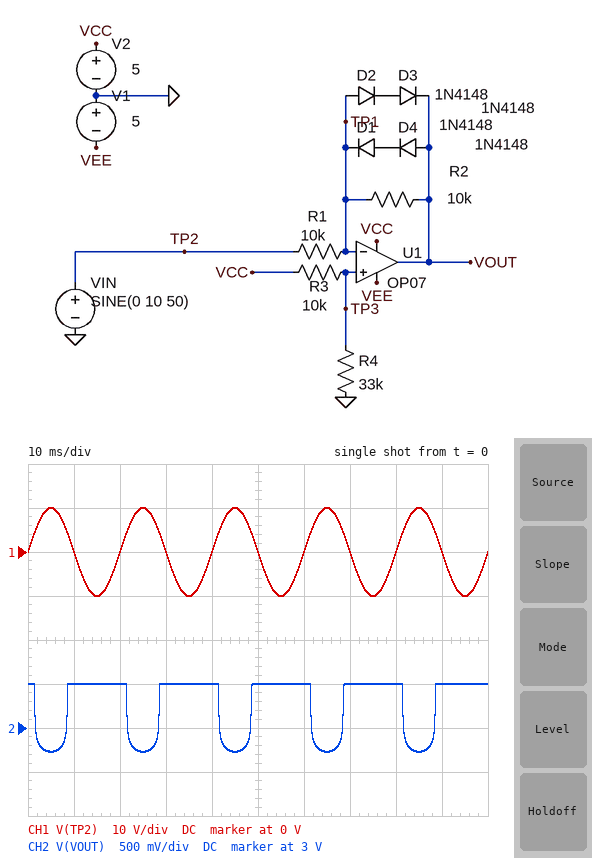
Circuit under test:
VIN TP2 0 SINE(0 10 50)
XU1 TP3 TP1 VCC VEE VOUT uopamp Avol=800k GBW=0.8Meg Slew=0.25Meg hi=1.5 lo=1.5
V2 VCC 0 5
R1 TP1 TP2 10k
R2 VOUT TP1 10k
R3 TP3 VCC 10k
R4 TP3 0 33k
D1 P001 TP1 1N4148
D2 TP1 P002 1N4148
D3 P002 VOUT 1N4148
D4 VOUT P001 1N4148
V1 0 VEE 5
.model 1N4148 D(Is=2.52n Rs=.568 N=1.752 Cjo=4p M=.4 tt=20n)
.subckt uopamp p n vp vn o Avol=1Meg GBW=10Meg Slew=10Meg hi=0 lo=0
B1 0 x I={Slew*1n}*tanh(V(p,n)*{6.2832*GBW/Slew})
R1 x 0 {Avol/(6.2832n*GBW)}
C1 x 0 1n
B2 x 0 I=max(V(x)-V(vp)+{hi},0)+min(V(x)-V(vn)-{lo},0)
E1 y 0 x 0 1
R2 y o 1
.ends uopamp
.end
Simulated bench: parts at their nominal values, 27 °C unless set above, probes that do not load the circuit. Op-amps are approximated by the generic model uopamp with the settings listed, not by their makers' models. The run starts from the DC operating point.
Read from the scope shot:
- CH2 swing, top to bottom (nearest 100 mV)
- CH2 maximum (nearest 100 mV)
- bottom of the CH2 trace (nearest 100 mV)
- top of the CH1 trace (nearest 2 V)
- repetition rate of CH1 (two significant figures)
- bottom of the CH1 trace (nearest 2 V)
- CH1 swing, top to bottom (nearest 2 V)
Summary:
800 mV
3.5 V
2.7 V
10 V
50 Hz
-10 V
20 V
